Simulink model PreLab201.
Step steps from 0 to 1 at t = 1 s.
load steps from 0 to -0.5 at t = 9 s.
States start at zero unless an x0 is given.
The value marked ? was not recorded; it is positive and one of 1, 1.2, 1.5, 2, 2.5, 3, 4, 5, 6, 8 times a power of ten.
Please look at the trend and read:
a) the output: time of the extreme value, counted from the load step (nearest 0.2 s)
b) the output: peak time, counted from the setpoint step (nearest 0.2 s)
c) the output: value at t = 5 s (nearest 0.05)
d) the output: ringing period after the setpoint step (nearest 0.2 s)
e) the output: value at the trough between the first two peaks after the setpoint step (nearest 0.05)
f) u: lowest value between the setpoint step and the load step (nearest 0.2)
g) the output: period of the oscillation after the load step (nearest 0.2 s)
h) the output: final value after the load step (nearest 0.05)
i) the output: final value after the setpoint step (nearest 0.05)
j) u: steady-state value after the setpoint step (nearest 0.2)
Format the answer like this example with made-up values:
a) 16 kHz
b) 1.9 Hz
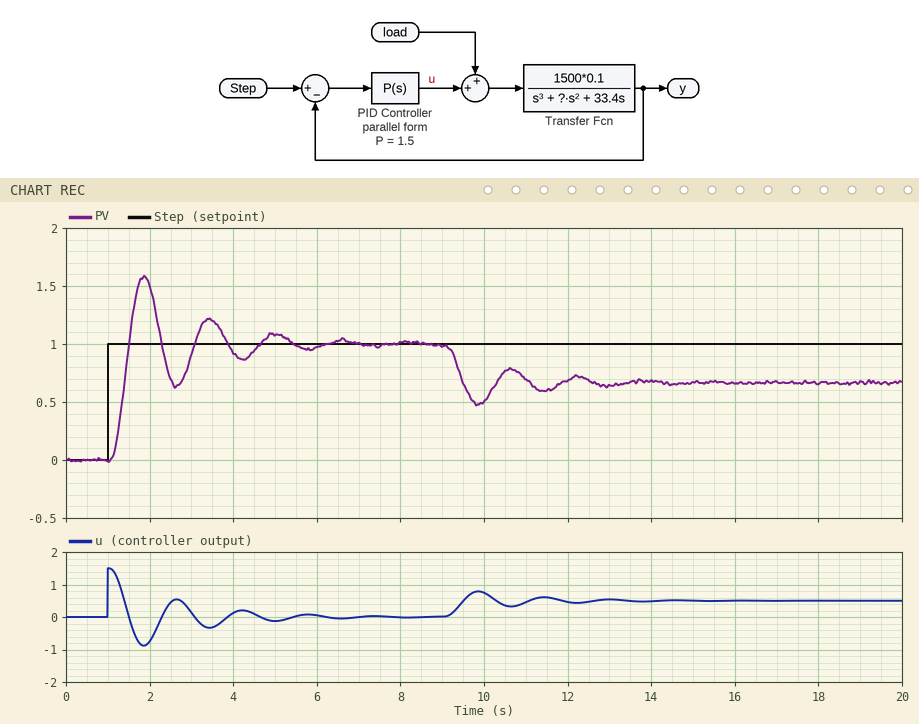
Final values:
a) 0.8 s
b) 0.8 s
c) 1.10
d) 1.6 s
e) 0.65
f) -0.8
g) 1.6 s
h) 0.65
i) 1.00
j) 0.0
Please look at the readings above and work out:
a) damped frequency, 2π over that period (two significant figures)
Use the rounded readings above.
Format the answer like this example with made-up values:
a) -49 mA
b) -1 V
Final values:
a) 3.9 rad/s
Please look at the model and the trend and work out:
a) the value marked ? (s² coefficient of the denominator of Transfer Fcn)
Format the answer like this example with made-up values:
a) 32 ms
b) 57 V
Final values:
a) 15
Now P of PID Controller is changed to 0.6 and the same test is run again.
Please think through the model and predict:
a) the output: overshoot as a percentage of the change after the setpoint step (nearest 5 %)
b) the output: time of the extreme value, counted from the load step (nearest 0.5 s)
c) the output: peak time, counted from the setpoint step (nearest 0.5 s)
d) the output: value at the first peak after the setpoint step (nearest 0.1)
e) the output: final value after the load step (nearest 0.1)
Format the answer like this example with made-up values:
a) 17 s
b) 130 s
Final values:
a) 25 %
b) 1.5 s
c) 1.5 s
d) 1.3
e) 0.2
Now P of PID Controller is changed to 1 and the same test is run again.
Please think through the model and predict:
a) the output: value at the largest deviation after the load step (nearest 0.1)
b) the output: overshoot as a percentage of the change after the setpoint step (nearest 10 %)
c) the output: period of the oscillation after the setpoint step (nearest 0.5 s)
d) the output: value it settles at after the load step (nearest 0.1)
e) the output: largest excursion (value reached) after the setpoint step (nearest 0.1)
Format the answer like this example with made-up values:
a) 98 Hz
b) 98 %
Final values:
a) 0.3
b) 40 %
c) 2.0 s
d) 0.5
e) 1.4
